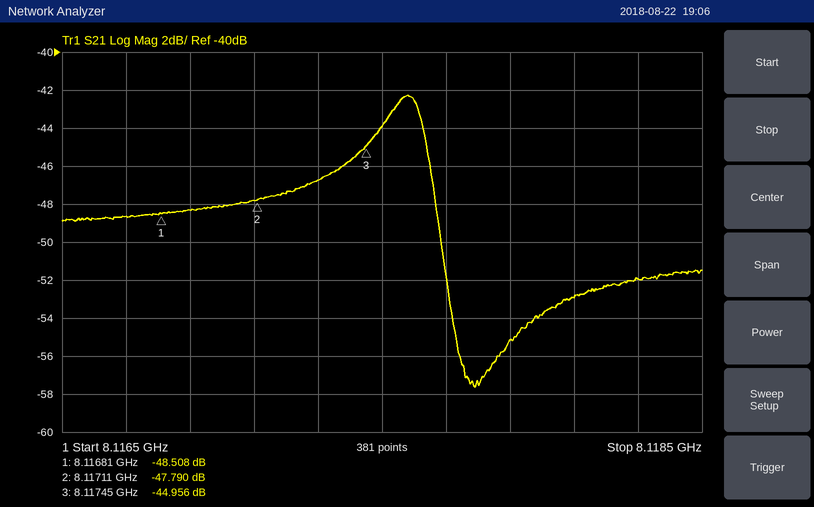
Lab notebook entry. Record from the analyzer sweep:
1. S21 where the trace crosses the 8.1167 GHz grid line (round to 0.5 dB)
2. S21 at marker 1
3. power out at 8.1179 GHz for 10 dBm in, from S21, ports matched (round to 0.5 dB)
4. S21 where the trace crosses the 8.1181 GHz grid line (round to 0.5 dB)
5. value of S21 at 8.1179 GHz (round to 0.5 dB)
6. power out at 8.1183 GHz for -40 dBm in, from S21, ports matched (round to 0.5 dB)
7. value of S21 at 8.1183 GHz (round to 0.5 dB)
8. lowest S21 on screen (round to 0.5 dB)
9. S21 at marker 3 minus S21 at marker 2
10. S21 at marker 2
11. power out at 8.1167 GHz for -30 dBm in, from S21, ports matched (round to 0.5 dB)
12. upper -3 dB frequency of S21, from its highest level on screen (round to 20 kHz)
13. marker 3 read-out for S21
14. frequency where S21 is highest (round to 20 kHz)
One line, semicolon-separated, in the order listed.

-48.5 dB; -48.508 dB; -45.0 dBm; -53.0 dB; -55.0 dB; -92.0 dBm; -52.0 dB; -57.5 dB; 2.834 dB; -47.790 dB; -78.5 dBm; 8.11764 GHz; -44.956 dB; 8.11758 GHz
